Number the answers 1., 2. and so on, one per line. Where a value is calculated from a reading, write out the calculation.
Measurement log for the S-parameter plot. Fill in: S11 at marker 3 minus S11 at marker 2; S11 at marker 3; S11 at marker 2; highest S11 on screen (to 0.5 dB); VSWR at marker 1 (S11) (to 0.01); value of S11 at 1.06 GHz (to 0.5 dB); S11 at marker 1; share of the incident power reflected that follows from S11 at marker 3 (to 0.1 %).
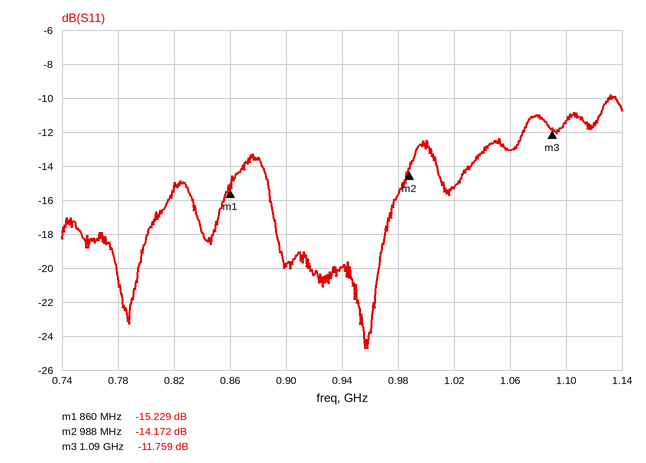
1. -11.759 − (-14.172) = 2.413 dB
2. -11.759 dB
3. -14.172 dB
4. -10.0 dB
5. (1 + 0.1732)/(1 − 0.1732) ≈ 1.42
6. -13.0 dB
7. -15.229 dB
8. 10^(-11.759/10) ≈ 6.7 %
